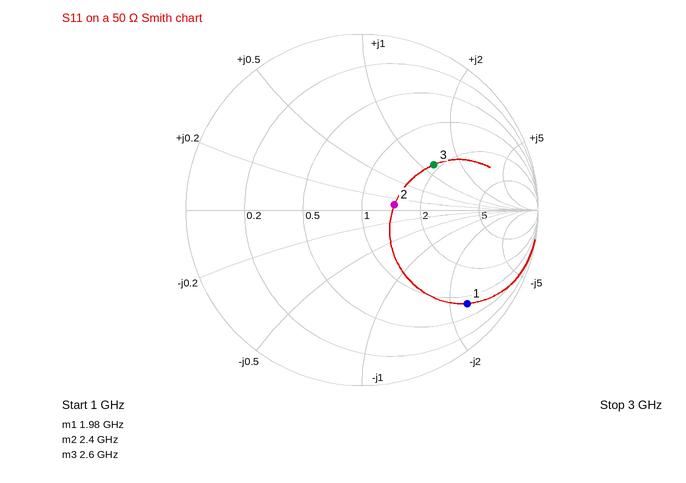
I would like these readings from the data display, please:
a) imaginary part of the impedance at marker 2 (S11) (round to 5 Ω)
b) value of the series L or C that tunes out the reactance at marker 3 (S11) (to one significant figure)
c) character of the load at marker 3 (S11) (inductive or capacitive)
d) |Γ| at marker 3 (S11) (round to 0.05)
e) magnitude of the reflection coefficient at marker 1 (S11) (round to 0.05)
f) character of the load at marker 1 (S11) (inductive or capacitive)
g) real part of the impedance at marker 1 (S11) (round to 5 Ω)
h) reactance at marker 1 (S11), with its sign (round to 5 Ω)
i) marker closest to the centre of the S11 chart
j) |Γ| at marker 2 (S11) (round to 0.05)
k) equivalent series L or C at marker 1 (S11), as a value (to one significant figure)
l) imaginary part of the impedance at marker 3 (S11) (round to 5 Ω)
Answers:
+5 Ω
1.0 pF
inductive
0.50
0.80
capacitive
40 Ω
-120 Ω
marker 2
0.20
700 fF
+60 Ω
